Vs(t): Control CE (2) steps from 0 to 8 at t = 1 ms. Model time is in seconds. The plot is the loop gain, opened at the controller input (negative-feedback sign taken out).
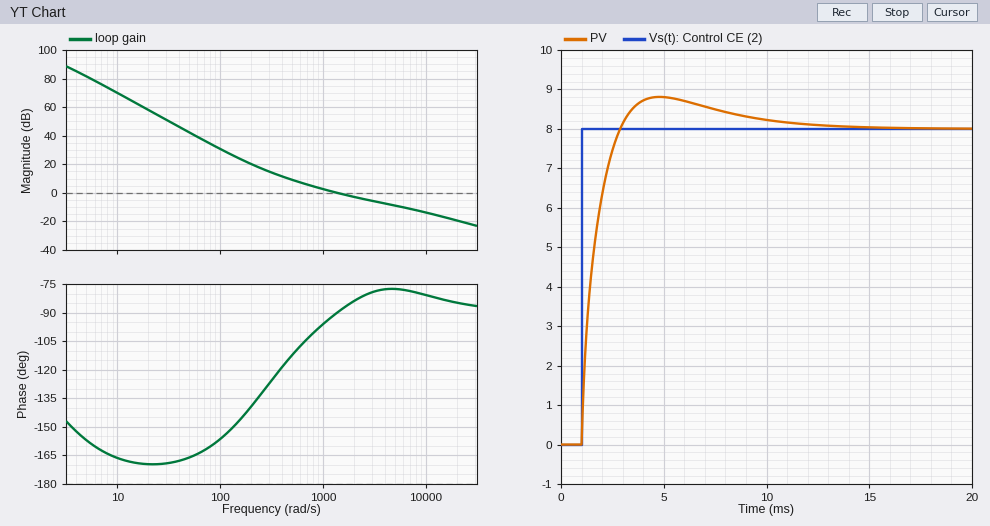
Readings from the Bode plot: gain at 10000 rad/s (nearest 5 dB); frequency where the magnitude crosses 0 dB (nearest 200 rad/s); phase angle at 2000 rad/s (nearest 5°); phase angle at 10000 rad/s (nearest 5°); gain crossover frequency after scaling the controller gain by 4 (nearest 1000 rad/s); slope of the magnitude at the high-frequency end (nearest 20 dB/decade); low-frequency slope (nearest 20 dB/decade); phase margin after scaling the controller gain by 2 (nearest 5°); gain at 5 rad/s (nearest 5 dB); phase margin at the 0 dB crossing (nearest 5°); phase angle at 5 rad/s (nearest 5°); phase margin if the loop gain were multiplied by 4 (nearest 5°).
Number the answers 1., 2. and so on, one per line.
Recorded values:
1. -15 dB
2. 1400 rad/s
3. -85°
4. -80°
5. 8000 rad/s
6. -20 dB/decade
7. -40 dB/decade
8. 100°
9. 80 dB
10. 90°
11. -155°
12. 100°
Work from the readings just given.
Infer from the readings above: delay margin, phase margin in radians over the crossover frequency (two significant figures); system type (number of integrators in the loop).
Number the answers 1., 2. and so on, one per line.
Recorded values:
1. 0.0011 s
2. 2
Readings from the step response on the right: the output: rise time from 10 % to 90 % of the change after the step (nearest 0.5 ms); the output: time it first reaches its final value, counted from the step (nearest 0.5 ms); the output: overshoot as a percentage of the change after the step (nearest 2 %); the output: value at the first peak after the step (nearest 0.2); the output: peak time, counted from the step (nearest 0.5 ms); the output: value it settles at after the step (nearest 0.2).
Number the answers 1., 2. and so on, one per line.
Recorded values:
1. 1.5 ms
2. 2.0 ms
3. 10 %
4. 8.8
5. 4.0 ms
6. 8.0
